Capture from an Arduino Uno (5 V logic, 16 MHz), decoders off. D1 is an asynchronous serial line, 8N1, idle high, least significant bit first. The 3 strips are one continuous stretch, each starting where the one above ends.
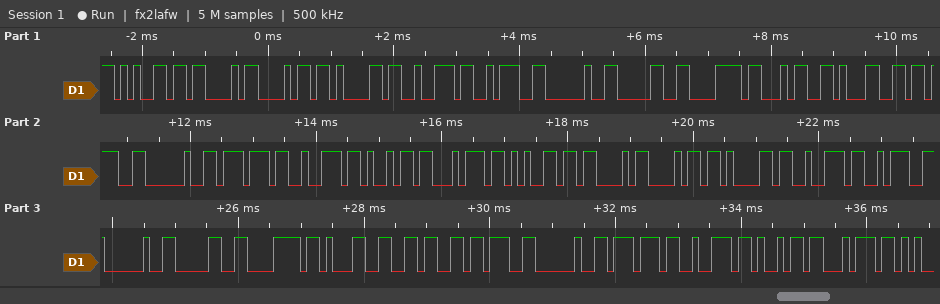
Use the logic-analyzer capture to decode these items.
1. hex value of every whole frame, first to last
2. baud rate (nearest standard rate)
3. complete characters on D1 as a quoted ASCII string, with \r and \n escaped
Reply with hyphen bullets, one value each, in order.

- 0x65 0x43 0x68 0x61 0x72 0x3A 0x20 0x30 0x78 0x34 0x31 0x3B 0x20 0x77 0x72 0x69 0x74 0x65 0x43 0x68 0x61 0x72 0x3A 0x20 0x30 0x78 0x31 0x36 0x3B 0x20 0x77 0x72 0x69 0x74
- 9600 baud
- "eChar: 0x41; writeChar: 0x16; writ"
